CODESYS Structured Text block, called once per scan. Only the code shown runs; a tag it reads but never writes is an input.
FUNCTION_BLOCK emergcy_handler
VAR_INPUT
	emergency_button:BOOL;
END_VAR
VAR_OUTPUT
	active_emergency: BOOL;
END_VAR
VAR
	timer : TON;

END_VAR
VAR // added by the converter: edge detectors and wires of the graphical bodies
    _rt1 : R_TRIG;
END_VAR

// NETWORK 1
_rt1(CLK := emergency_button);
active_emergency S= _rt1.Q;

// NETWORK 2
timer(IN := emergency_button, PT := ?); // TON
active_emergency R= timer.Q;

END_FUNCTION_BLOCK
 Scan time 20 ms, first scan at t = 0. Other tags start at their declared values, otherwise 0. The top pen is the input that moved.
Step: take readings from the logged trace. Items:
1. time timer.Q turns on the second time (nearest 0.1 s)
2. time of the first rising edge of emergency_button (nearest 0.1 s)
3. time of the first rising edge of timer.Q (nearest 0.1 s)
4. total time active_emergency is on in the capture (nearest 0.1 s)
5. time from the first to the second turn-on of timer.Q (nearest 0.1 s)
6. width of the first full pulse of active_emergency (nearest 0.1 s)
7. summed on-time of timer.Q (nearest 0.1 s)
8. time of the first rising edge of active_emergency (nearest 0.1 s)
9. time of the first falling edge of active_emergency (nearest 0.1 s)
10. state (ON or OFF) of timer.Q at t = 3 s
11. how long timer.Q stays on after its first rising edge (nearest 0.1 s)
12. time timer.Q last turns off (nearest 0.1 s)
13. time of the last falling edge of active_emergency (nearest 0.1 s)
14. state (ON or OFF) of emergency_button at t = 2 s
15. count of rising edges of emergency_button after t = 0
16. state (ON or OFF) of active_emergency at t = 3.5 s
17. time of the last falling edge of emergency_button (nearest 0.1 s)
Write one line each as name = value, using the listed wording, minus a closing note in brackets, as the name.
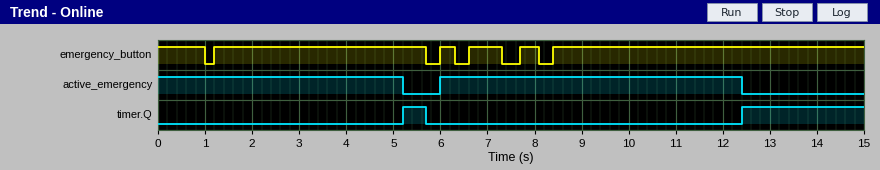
time timer.Q turns on the second time = 12.4 s
time of the first rising edge of emergency_button = 1.2 s
time of the first rising edge of timer.Q = 5.2 s
total time active_emergency is on in the capture = 11.6 s
time from the first to the second turn-on of timer.Q = 7.2 s
width of the first full pulse of active_emergency = 6.4 s
summed on-time of timer.Q = 3.1 s
time of the first rising edge of active_emergency = 6.0 s
time of the first falling edge of active_emergency = 5.2 s
state (ON or OFF) of timer.Q at t = 3 s = OFF
how long timer.Q stays on after its first rising edge = 0.5 s
time timer.Q last turns off = 5.7 s
time of the last falling edge of active_emergency = 12.4 s
state (ON or OFF) of emergency_button at t = 2 s = ON
count of rising edges of emergency_button after t = 0 = 5
state (ON or OFF) of active_emergency at t = 3.5 s = ON
time of the last falling edge of emergency_button = 8.1 s
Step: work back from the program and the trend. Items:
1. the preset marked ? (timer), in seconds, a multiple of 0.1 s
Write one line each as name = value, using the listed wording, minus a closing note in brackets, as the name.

the preset marked ? (timer), in seconds, a multiple of 0.1 s = 4.0 s
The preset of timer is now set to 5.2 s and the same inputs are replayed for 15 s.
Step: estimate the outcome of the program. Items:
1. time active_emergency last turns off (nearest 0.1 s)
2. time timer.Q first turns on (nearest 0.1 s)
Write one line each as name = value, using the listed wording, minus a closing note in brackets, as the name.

time active_emergency last turns off = 13.6 s
time timer.Q first turns on = 13.6 s
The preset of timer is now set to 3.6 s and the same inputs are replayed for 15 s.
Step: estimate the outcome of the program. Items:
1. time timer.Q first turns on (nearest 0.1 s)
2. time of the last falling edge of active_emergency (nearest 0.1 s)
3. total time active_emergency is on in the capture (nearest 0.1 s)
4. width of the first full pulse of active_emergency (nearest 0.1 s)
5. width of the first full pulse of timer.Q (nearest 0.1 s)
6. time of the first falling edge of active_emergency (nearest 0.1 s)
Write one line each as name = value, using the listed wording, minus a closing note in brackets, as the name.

time timer.Q first turns on = 4.8 s
time of the last falling edge of active_emergency = 12.0 s
total time active_emergency is on in the capture = 10.8 s
width of the first full pulse of active_emergency = 6.0 s
width of the first full pulse of timer.Q = 0.9 s
time of the first falling edge of active_emergency = 4.8 s
